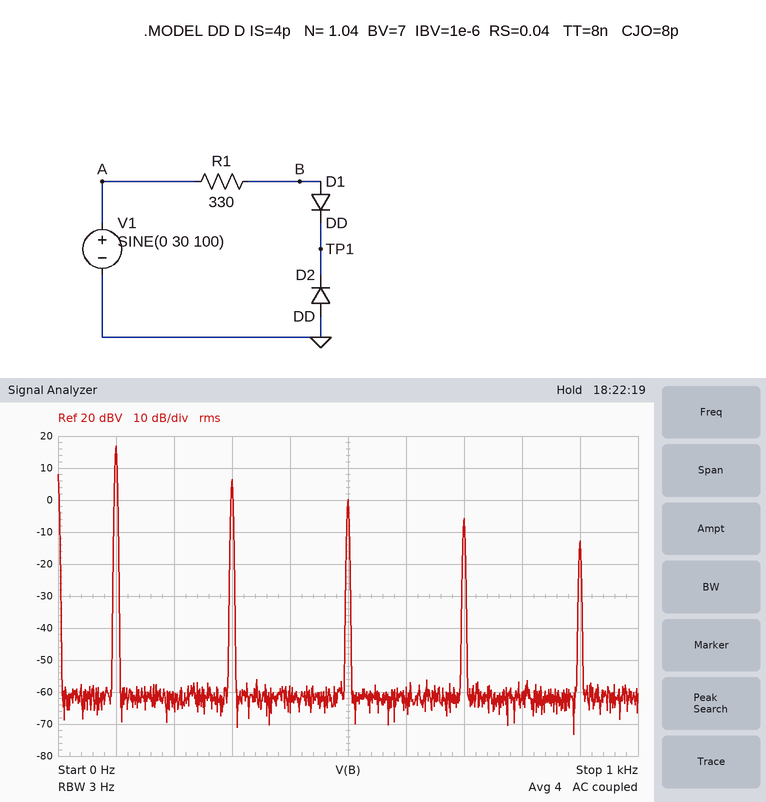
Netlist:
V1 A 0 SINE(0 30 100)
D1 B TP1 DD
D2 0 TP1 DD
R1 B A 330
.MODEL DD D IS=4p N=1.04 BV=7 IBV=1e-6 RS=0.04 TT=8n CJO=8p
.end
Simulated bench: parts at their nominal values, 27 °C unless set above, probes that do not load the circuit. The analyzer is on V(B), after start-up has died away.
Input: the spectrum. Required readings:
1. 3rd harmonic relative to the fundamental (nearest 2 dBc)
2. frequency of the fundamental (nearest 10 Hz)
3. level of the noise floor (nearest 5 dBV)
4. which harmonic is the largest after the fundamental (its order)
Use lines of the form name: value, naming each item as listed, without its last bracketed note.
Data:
3rd harmonic relative to the fundamental: -10 dBc
frequency of the fundamental: 100 Hz
level of the noise floor: -60 dBV
which harmonic is the largest after the fundamental: 3
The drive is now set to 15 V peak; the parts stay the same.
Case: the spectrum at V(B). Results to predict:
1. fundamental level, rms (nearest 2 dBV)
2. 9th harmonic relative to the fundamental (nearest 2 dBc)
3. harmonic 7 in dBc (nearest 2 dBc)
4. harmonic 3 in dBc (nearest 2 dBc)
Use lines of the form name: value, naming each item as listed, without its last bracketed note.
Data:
fundamental level, rms: 16 dBV
9th harmonic relative to the fundamental: -34 dBc
harmonic 7 in dBc: -34 dBc
harmonic 3 in dBc: -14 dBc
